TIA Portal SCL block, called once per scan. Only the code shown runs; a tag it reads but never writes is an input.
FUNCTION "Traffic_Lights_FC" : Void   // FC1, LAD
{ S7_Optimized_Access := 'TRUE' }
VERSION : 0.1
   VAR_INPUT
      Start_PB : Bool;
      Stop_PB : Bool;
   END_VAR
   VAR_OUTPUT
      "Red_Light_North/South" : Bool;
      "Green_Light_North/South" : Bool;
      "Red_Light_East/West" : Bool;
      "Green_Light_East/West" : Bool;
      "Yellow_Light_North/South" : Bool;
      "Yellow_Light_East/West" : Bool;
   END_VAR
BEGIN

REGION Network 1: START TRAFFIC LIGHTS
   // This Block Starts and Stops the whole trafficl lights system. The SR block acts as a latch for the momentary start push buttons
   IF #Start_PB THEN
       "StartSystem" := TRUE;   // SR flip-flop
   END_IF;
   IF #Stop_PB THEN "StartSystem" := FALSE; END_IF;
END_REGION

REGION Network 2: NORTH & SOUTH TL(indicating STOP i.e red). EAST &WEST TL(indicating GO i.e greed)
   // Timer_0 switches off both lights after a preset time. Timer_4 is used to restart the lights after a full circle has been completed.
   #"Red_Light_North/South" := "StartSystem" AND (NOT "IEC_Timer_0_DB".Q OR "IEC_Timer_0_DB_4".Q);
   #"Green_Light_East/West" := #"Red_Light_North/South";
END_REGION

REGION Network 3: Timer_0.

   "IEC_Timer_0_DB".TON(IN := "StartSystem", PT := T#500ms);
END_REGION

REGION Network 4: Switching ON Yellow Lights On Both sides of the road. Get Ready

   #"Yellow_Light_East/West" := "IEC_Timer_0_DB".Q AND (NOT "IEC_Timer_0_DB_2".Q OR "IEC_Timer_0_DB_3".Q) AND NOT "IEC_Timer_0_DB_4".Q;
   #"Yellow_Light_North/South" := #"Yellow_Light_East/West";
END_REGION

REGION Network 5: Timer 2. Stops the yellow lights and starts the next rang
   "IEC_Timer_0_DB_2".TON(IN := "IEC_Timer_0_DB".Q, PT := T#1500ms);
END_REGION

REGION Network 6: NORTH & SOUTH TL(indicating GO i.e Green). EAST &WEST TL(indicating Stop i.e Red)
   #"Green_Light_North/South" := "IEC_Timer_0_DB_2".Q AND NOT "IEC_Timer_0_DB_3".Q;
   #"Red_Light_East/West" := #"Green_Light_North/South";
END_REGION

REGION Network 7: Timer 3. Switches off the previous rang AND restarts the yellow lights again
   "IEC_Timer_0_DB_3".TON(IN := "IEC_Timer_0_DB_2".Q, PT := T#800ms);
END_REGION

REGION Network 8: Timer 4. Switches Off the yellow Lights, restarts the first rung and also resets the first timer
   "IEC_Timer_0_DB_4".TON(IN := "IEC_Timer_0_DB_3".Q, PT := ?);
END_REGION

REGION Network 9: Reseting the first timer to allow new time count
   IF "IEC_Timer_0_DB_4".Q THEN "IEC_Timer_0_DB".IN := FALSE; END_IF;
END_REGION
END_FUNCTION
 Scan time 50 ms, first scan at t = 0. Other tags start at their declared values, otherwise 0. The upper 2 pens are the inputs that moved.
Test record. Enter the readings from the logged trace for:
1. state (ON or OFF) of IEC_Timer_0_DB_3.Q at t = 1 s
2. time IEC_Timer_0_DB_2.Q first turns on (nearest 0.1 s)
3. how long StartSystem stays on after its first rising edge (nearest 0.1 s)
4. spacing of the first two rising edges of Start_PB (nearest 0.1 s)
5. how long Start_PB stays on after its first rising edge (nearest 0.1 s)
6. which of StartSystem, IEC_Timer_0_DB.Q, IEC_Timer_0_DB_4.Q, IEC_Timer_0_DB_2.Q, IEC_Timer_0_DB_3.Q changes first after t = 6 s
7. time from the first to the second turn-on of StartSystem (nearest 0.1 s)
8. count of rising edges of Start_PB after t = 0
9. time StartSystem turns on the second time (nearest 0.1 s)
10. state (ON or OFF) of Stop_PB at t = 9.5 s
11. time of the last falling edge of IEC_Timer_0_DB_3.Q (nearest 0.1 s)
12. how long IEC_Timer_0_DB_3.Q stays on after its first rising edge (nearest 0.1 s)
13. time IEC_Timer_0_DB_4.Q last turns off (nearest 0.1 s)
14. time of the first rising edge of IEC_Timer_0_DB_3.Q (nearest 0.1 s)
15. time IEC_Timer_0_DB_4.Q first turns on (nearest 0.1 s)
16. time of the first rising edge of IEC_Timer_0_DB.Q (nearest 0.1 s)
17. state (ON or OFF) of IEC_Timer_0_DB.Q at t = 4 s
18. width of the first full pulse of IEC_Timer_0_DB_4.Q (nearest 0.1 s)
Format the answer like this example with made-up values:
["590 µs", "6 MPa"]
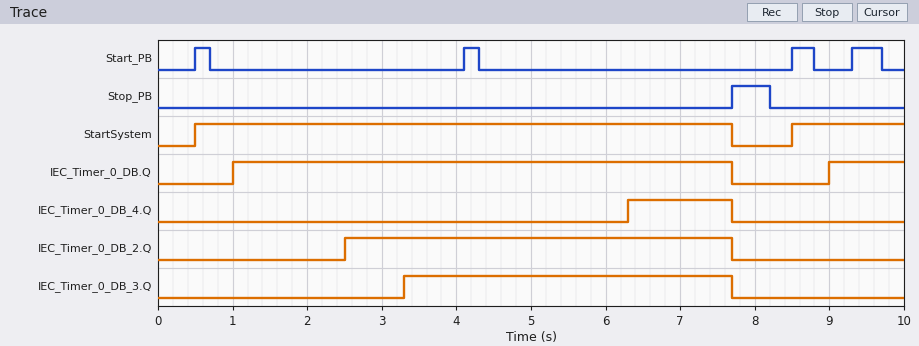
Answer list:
["OFF", "2.5 s", "7.2 s", "3.6 s", "0.2 s", "IEC_Timer_0_DB_4.Q", "8.0 s", "4", "8.5 s", "OFF", "7.7 s", "4.4 s", "7.7 s", "3.3 s", "6.3 s", "1.0 s", "ON", "1.4 s"]
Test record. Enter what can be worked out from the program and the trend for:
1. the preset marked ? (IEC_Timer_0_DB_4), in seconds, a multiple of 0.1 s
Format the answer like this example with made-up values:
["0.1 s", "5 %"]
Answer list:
["3.0 s"]
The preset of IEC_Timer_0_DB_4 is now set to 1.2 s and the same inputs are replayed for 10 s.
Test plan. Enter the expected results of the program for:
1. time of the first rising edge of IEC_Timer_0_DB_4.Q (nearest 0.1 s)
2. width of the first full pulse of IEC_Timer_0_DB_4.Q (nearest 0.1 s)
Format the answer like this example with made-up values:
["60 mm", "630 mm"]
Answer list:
["4.5 s", "3.2 s"]
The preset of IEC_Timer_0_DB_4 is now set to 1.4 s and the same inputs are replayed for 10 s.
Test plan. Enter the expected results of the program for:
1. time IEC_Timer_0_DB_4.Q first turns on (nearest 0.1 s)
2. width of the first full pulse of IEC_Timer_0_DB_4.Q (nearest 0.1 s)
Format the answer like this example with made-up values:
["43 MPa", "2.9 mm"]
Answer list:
["4.7 s", "3.0 s"]
